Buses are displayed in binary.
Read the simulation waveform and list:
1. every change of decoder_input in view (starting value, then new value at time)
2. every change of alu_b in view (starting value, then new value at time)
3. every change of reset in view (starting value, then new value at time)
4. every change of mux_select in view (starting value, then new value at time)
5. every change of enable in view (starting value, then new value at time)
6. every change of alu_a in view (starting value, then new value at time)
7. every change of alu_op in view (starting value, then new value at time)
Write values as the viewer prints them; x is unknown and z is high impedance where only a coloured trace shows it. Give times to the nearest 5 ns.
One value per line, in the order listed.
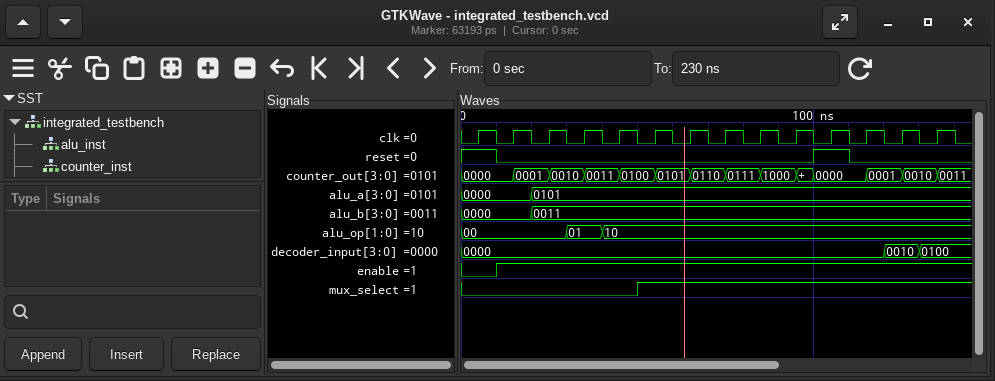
0000, 0010 at 120 ns, 0100 at 130 ns
0000, 0011 at 20 ns
1, 0 at 10 ns, 1 at 100 ns, 0 at 110 ns
0, 1 at 50 ns
0, 1 at 10 ns
0000, 0101 at 20 ns
00, 01 at 30 ns, 10 at 40 ns
